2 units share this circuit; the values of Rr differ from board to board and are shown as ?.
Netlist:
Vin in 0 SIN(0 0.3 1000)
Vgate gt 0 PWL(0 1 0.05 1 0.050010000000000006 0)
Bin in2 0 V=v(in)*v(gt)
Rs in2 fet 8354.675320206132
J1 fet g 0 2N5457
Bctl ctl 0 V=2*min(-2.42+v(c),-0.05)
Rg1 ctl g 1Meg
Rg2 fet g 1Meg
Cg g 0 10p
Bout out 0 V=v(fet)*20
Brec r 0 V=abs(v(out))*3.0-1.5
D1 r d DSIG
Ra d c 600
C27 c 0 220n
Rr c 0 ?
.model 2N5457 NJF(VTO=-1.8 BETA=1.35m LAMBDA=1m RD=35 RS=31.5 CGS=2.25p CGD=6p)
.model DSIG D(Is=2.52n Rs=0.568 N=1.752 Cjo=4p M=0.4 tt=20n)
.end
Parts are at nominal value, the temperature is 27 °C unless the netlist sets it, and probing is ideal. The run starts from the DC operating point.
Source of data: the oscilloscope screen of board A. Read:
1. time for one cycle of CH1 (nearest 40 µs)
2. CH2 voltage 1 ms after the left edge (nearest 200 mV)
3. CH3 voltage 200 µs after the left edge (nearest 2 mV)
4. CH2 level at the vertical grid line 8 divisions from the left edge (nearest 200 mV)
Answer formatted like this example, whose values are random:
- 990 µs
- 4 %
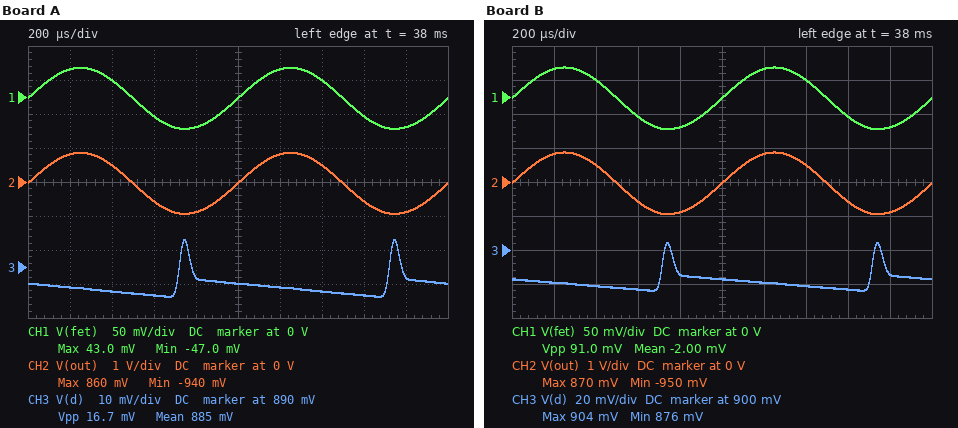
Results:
- 1.00 ms
- 0 V
- 884 mV
- -600 mV
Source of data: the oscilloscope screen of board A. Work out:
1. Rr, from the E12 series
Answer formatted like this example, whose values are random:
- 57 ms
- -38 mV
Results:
- 680 kΩ
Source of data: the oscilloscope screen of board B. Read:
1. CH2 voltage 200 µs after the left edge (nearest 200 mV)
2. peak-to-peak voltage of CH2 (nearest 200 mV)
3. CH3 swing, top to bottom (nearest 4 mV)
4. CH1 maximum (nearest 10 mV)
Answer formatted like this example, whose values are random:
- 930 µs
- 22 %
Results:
- 800 mV
- 1.8 V
- 28 mV
- 40 mV
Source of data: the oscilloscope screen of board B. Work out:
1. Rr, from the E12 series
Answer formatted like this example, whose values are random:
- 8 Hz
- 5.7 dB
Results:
- 390 kΩ
